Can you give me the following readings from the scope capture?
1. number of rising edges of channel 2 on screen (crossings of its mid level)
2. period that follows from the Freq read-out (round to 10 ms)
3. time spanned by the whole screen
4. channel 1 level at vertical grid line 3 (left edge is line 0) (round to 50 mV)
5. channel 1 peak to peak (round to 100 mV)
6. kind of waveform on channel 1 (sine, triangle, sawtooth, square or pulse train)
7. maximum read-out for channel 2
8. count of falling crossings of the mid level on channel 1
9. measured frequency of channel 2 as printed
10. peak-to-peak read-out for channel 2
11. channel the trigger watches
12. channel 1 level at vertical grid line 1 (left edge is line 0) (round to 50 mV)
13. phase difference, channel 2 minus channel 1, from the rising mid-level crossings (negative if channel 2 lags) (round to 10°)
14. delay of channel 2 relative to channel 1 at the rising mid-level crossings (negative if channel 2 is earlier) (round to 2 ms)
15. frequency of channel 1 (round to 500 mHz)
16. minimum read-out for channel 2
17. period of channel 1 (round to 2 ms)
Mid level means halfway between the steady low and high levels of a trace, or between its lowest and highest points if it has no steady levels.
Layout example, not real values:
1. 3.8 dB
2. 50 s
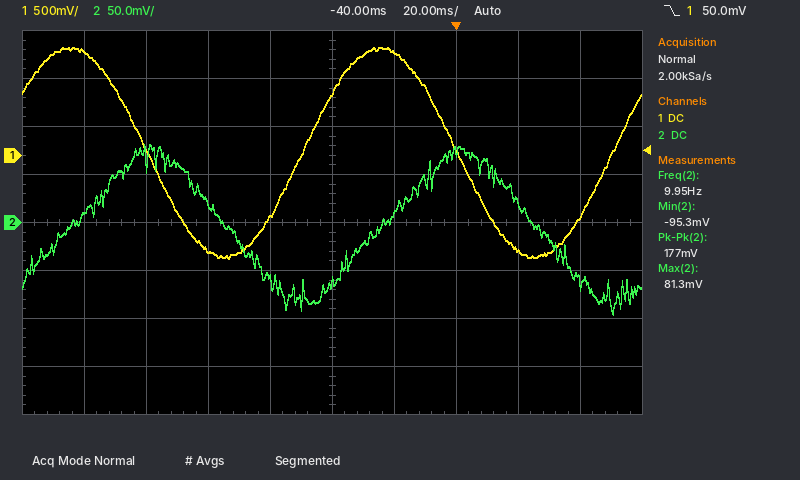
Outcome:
1. 2
2. 100 ms
3. 200 ms
4. -1.00 V
5. 2.20 V
6. sine
7. 81.3 mV
8. 2
9. 9.95 Hz
10. 177 mV
11. channel 1
12. 1.10 V
13. -90°
14. +24 ms
15. 10.0 Hz
16. -95.3 mV
17. 100 ms
